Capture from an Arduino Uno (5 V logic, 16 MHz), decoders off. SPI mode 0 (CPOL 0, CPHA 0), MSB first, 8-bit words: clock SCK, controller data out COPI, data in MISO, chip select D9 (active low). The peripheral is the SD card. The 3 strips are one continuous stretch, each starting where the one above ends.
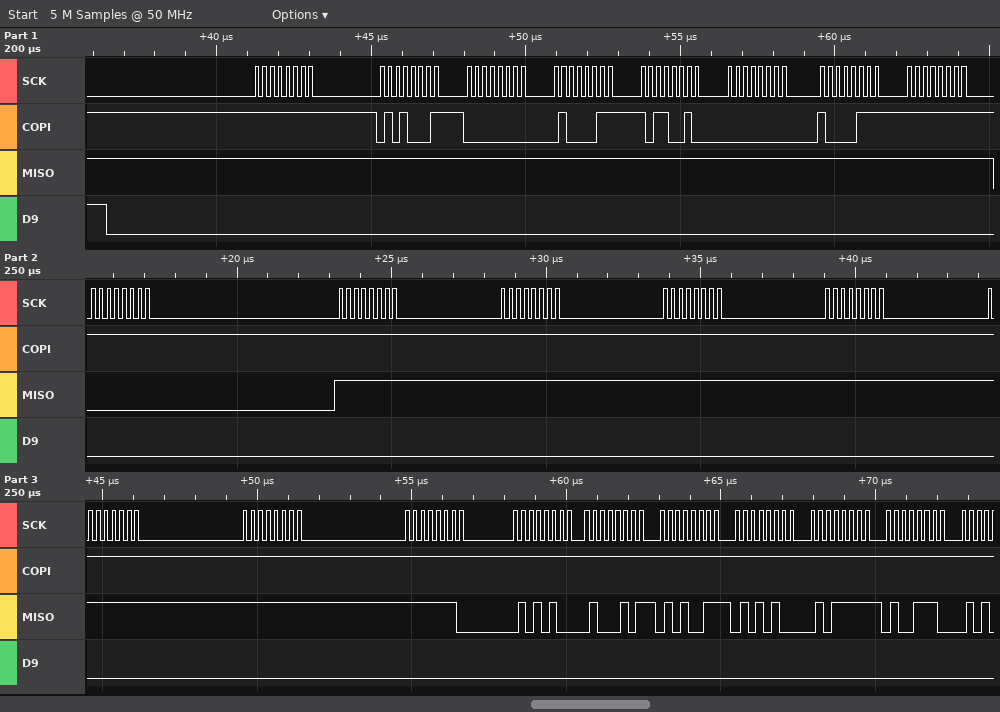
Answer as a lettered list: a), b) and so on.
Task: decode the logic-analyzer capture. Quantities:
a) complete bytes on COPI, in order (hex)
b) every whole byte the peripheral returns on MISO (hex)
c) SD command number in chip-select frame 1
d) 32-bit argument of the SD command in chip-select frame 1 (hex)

a) FF 51 00 43 B2 00 87 FF FF FF FF FF FF FF FF FF FF FF FF FF FF FF
b) FF FF FF FF FF FF FF FF 00 FF FF FF FF FF FF FE 54 45 53 54 5F 4E
c) CMD17
d) 0x0043B200
